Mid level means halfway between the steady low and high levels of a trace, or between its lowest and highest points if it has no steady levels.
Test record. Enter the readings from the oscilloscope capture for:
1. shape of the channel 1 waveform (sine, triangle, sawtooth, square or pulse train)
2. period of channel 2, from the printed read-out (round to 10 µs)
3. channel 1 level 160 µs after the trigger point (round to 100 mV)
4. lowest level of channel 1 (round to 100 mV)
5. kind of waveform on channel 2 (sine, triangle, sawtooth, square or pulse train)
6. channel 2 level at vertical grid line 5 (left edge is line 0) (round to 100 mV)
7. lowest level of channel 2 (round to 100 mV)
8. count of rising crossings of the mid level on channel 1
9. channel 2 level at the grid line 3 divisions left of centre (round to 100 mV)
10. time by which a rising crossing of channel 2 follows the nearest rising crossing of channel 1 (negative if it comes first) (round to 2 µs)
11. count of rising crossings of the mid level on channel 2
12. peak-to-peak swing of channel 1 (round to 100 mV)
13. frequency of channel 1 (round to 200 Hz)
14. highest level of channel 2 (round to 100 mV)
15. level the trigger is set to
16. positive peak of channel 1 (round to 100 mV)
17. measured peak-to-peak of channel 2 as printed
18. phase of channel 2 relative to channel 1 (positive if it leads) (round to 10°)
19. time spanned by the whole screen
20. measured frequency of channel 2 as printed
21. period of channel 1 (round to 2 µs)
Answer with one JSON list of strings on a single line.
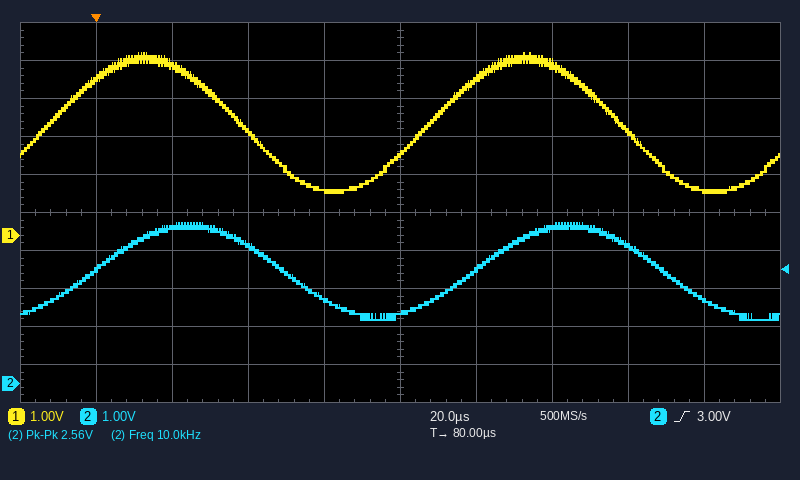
["sine", "100 µs", "1.2 V", "1.1 V", "sine", "1.9 V", "1.7 V", "2", "4.1 V", "+12 µs", "2", "3.7 V", "10.0 kHz", "4.2 V", "3.00 V", "4.8 V", "2.56 V", "-40°", "200 µs", "10.0 kHz", "100 µs"]
